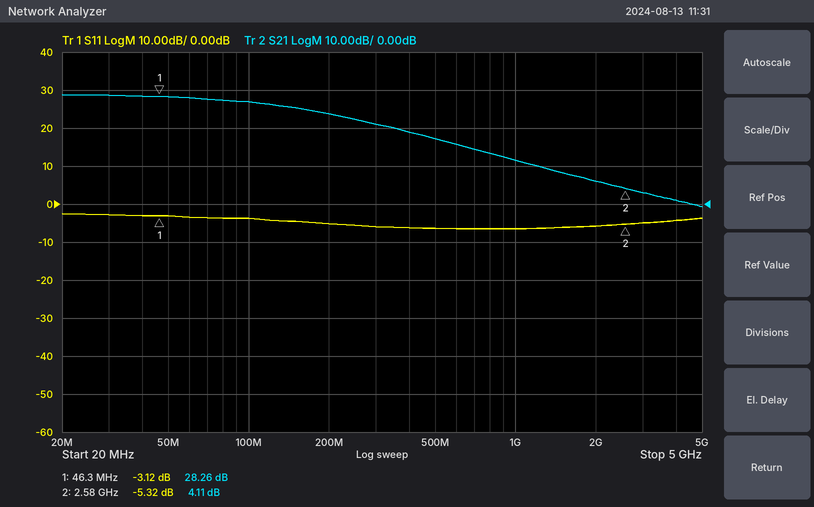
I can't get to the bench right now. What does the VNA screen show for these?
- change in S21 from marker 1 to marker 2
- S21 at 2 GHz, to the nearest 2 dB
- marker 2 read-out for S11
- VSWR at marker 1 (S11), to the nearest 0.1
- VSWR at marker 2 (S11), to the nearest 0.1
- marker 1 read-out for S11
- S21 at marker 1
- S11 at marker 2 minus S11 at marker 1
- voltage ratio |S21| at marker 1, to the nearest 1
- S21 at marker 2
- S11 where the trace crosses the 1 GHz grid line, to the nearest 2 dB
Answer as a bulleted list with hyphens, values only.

- -24.15 dB
- 6 dB
- -5.32 dB
- 5.6
- 3.4
- -3.12 dB
- 28.26 dB
- -2.20 dB
- 26
- 4.11 dB
- -6 dB
